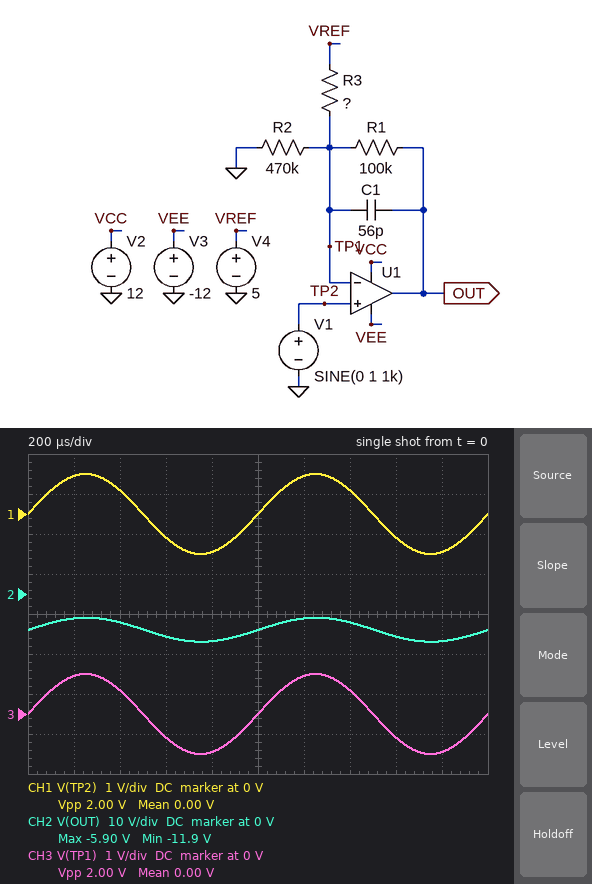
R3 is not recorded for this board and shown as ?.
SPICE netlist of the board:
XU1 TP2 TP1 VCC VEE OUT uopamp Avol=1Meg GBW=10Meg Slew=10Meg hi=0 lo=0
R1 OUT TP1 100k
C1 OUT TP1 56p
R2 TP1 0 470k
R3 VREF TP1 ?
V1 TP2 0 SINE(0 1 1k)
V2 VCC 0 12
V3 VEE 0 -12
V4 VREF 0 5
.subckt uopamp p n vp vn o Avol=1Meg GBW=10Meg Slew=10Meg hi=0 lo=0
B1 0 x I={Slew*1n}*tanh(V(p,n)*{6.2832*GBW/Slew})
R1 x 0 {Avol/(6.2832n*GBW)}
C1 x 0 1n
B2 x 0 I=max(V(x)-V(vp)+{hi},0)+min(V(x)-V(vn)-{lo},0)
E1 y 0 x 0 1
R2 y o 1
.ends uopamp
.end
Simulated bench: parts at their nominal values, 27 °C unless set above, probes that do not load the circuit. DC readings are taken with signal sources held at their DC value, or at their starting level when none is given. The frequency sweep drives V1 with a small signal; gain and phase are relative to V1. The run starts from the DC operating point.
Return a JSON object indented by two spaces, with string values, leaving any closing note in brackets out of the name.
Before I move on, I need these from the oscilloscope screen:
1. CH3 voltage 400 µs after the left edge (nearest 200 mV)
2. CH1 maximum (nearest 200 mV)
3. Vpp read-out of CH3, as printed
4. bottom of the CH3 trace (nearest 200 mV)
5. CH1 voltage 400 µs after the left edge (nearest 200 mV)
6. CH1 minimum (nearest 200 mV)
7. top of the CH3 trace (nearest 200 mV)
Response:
{
  "CH3 voltage 400 µs after the left edge": "600 mV",
  "CH1 maximum": "1.0 V",
  "Vpp read-out of CH3, as printed": "2.00 V",
  "bottom of the CH3 trace": "-1.0 V",
  "CH1 voltage 400 µs after the left edge": "600 mV",
  "CH1 minimum": "-1.0 V",
  "top of the CH3 trace": "1.0 V"
}
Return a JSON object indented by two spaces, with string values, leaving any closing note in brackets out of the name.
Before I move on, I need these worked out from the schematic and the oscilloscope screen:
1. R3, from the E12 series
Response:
{
  "R3, from the E12 series": "56 kΩ"
}
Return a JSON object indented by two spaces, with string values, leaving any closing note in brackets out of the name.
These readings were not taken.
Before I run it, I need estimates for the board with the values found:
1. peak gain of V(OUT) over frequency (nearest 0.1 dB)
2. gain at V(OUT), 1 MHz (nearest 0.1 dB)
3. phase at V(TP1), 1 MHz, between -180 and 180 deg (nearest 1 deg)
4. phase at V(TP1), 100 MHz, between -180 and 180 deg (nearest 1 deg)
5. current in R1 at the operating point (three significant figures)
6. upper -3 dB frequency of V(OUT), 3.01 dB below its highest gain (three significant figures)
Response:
{
  "peak gain of V(OUT) over frequency": "9.5 dB",
  "gain at V(OUT), 1 MHz": "-0.1 dB",
  "phase at V(TP1), 1 MHz, between -180 and 180 deg": "-6 deg",
  "phase at V(TP1), 100 MHz, between -180 and 180 deg": "-84 deg",
  "current in R1 at the operating point": "89.3 µA",
  "upper -3 dB frequency of V(OUT), 3.01 dB below its highest gain": "32.0 kHz"
}
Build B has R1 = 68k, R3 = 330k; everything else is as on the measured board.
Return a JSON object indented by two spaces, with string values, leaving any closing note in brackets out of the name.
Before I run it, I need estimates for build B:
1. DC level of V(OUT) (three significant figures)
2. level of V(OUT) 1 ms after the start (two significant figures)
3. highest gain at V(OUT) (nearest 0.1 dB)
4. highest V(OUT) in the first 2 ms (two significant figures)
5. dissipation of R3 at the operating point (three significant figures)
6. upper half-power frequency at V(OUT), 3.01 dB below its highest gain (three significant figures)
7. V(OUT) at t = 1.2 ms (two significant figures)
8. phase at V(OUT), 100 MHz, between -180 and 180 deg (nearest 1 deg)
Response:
{
  "DC level of V(OUT)": "-1.03 V",
  "level of V(OUT) 1 ms after the start": "-1.0 V",
  "highest gain at V(OUT)": "2.6 dB",
  "highest V(OUT) in the first 2 ms": "320 mV",
  "dissipation of R3 at the operating point": "75.8 µW",
  "upper half-power frequency at V(OUT), 3.01 dB below its highest gain": "3.06 MHz",
  "V(OUT) at t = 1.2 ms": "250 mV",
  "phase at V(OUT), 100 MHz, between -180 and 180 deg": "-84 deg"
}
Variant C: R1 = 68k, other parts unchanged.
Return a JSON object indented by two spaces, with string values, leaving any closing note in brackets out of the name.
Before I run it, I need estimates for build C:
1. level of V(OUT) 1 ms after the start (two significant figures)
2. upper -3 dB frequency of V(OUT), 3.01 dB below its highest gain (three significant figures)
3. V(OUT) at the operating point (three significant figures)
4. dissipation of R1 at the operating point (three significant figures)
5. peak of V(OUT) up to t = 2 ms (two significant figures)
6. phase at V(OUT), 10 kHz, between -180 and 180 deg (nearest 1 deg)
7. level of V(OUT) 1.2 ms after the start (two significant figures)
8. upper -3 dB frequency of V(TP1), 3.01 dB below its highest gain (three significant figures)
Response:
{
  "level of V(OUT) 1 ms after the start": "-6.1 V",
  "upper -3 dB frequency of V(OUT), 3.01 dB below its highest gain": "51.8 kHz",
  "V(OUT) at the operating point": "-6.07 V",
  "dissipation of R1 at the operating point": "542 µW",
  "peak of V(OUT) up to t = 2 ms": "-3.7 V",
  "phase at V(OUT), 10 kHz, between -180 and 180 deg": "-8 deg",
  "level of V(OUT) 1.2 ms after the start": "-3.8 V",
  "upper -3 dB frequency of V(TP1), 3.01 dB below its highest gain": "9.94 MHz"
}
